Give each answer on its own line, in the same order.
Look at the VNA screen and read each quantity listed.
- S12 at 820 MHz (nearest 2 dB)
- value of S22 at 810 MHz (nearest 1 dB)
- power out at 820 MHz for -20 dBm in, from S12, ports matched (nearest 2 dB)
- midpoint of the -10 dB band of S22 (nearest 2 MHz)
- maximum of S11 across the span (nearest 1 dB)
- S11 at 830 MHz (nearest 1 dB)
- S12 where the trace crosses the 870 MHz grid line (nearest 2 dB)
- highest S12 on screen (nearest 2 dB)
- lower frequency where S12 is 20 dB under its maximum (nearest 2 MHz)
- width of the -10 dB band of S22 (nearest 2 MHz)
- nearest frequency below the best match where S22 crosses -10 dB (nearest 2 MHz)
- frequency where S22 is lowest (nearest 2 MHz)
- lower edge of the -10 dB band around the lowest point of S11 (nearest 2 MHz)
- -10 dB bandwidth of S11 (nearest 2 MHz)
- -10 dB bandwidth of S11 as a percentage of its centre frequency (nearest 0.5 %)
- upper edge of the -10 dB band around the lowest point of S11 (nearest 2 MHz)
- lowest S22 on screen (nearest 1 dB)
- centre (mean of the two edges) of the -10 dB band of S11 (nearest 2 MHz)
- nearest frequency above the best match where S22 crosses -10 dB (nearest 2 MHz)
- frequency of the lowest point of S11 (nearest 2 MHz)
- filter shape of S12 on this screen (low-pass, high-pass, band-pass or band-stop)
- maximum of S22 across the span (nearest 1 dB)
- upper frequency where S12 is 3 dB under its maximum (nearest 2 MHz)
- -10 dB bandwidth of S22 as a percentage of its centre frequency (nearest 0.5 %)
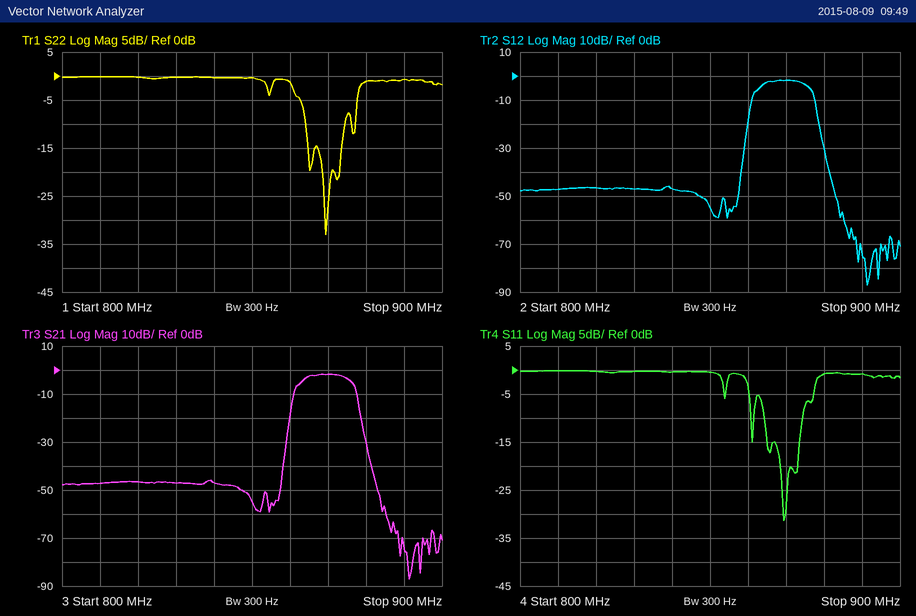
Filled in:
-46 dB
0 dB
-66 dBm
870 MHz
0 dB
0 dB
-2 dB
-2 dB
860 MHz
10 MHz
864 MHz
870 MHz
864 MHz
10 MHz
1.0 %
874 MHz
-33 dB
870 MHz
874 MHz
870 MHz
band-pass
0 dB
876 MHz
1.0 %
